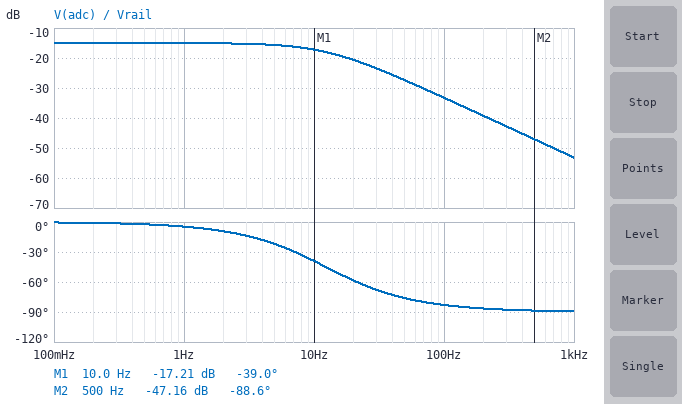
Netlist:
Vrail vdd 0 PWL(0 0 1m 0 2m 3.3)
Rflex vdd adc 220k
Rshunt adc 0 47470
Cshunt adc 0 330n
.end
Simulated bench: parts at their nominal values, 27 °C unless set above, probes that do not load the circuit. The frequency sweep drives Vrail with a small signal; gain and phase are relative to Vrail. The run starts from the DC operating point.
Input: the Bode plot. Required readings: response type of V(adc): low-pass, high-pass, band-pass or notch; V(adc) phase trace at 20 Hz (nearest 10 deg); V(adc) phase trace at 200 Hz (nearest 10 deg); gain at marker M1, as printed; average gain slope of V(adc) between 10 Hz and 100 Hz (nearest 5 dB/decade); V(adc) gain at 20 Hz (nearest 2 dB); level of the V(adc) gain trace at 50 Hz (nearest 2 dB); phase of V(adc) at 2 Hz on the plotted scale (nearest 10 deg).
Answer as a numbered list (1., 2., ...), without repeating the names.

1. low-pass
2. -60 deg
3. -90 deg
4. -17.21 dB
5. -15 dB/decade
6. -20 dB
7. -28 dB
8. -10 deg
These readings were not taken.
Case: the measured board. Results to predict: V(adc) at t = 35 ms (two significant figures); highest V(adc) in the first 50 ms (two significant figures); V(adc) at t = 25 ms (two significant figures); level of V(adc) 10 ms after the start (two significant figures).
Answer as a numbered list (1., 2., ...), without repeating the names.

1. 540 mV
2. 570 mV
3. 490 mV
4. 280 mV
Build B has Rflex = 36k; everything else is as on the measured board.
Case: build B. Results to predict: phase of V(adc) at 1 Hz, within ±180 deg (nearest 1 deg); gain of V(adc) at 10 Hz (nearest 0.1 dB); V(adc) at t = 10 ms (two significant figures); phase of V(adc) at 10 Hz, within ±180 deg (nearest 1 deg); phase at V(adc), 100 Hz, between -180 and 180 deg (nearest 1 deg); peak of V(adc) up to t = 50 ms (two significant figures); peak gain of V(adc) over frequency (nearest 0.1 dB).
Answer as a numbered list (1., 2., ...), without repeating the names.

1. -2 deg
2. -5.6 dB
3. 1.3 V
4. -23 deg
5. -77 deg
6. 1.9 V
7. -4.9 dB
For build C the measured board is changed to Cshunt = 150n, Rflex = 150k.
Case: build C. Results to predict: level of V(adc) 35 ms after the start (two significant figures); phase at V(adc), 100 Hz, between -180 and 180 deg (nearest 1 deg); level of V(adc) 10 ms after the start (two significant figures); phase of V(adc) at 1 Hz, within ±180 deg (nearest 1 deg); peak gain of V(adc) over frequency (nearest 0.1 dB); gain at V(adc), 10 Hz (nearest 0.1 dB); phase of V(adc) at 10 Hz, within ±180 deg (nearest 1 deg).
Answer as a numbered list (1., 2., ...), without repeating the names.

1. 790 mV
2. -74 deg
3. 630 mV
4. -2 deg
5. -12.4 dB
6. -12.9 dB
7. -19 deg
